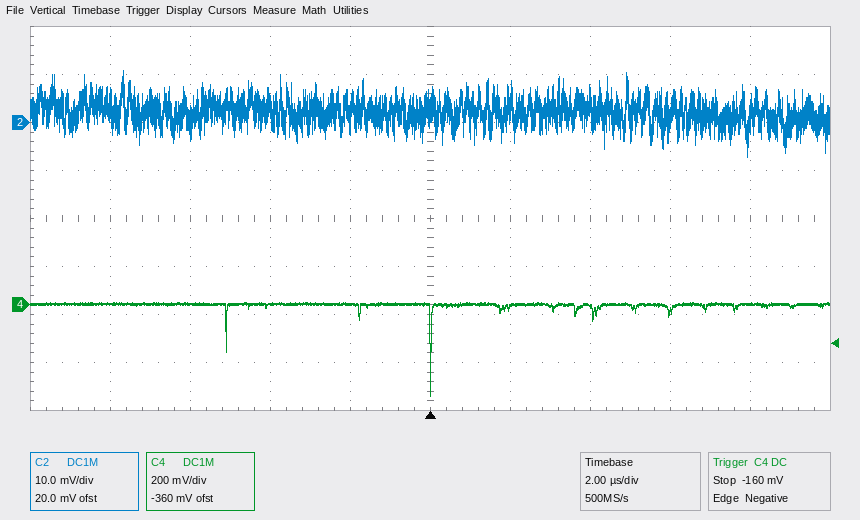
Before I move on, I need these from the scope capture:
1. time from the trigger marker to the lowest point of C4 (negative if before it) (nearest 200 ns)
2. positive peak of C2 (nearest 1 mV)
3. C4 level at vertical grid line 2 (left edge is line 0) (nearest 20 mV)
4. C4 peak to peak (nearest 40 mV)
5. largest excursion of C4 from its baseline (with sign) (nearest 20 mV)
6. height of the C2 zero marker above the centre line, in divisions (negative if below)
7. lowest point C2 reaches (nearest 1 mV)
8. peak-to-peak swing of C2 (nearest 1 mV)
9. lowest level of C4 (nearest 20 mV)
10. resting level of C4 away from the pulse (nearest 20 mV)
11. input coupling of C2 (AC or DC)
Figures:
0.0 µs
11 mV
0 mV
400 mV
-380 mV
+2.0 div
-7 mV
18 mV
-380 mV
0 mV
DC
